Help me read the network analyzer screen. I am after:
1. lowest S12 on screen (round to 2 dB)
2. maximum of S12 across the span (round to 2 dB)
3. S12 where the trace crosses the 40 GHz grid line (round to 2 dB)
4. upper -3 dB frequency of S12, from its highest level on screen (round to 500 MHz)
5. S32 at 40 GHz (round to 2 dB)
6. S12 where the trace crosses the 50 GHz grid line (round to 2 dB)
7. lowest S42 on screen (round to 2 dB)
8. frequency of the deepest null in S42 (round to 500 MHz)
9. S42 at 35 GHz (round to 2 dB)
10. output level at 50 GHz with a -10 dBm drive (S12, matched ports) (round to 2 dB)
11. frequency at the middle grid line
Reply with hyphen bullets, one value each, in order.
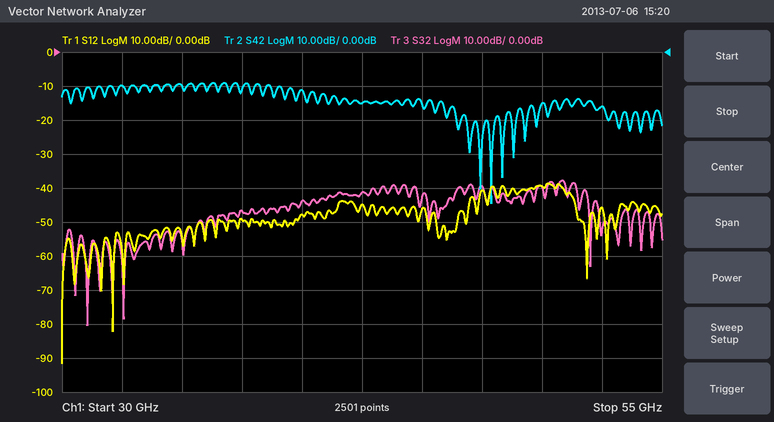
- -92 dB
- -38 dB
- -48 dB
- 51.0 GHz
- -44 dB
- -40 dB
- -44 dB
- 48.0 GHz
- -10 dB
- -50 dBm
- 42.5 GHz
